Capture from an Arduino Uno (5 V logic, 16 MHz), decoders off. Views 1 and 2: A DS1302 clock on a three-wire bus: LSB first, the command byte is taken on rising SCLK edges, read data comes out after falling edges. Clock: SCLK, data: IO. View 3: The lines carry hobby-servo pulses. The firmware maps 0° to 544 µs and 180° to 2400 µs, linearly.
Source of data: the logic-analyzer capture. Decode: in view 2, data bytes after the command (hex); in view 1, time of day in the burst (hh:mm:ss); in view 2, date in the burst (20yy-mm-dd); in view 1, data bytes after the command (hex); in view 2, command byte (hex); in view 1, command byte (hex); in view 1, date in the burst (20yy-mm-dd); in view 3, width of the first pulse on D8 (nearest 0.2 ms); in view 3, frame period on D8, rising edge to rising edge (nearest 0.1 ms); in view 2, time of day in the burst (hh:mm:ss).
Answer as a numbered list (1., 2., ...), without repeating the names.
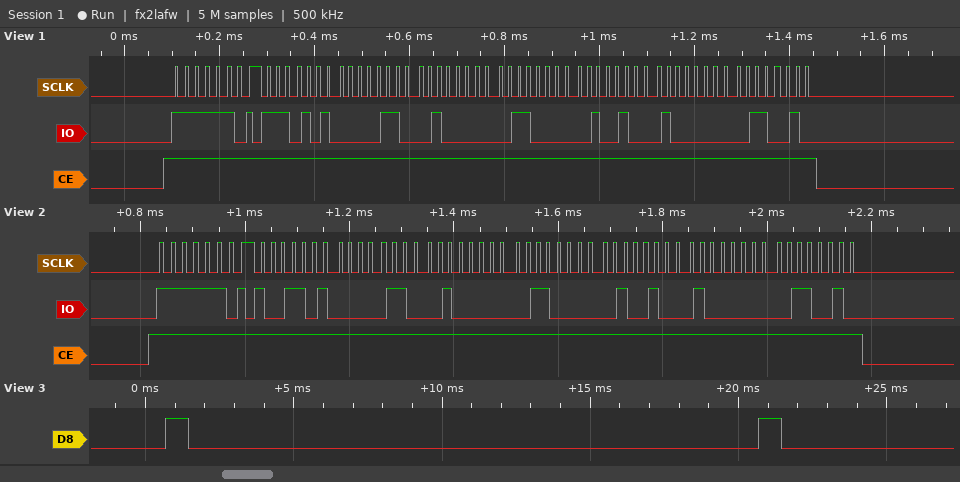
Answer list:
1. 59 30 02 06 12 01 26
2. 02:30:57
3. 2026-12-06
4. 57 30 02 06 12 01 26
5. 0xBF
6. 0xBF
7. 2026-12-06
8. 0.8 ms
9. 20.0 ms
10. 02:30:59
